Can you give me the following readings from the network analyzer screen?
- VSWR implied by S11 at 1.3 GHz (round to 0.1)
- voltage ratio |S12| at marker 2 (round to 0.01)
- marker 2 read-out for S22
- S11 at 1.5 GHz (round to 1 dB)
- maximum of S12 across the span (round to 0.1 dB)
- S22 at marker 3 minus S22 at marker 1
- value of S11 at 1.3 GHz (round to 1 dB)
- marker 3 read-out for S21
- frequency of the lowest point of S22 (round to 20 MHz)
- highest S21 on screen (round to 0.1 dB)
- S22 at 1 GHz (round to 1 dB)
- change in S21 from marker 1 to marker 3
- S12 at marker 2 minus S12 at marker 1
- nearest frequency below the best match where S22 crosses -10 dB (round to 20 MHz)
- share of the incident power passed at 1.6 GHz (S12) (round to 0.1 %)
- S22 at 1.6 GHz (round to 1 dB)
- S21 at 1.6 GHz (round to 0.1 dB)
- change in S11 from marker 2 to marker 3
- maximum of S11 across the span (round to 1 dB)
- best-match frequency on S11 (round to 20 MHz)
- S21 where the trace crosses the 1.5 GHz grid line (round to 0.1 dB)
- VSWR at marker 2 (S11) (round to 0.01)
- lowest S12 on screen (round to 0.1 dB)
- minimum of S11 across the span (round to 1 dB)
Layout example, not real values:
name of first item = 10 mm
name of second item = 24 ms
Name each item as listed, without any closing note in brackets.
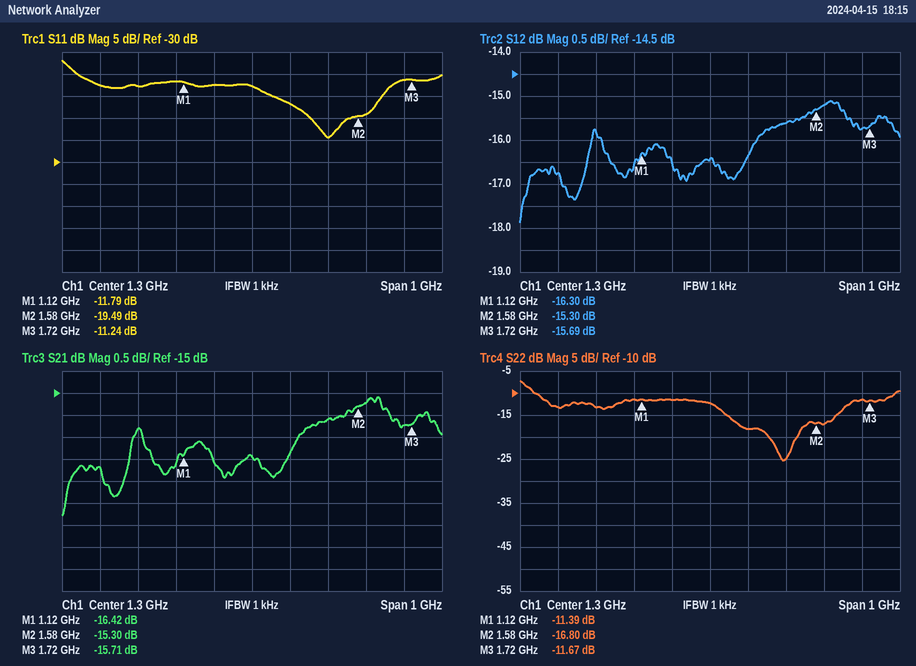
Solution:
VSWR implied by S11 at 1.3 GHz = 1.6
voltage ratio |S12| at marker 2 = 0.17
marker 2 read-out for S22 = -16.80 dB
S11 at 1.5 GHz = -24 dB
maximum of S12 across the span = -15.1 dB
S22 at marker 3 minus S22 at marker 1 = -0.28 dB
value of S11 at 1.3 GHz = -13 dB
marker 3 read-out for S21 = -15.71 dB
frequency of the lowest point of S22 = 1.50 GHz
highest S21 on screen = -15.1 dB
S22 at 1 GHz = -13 dB
change in S21 from marker 1 to marker 3 = 0.71 dB
S12 at marker 2 minus S12 at marker 1 = 1.00 dB
nearest frequency below the best match where S22 crosses -10 dB = 840 MHz
share of the incident power passed at 1.6 GHz (S12) = 3.0 %
S22 at 1.6 GHz = -17 dB
S21 at 1.6 GHz = -15.2 dB
change in S11 from marker 2 to marker 3 = 8.25 dB
maximum of S11 across the span = -7 dB
best-match frequency on S11 = 1.50 GHz
S21 where the trace crosses the 1.5 GHz grid line = -15.6 dB
VSWR at marker 2 (S11) = 1.24
lowest S12 on screen = -17.9 dB
minimum of S11 across the span = -24 dB
